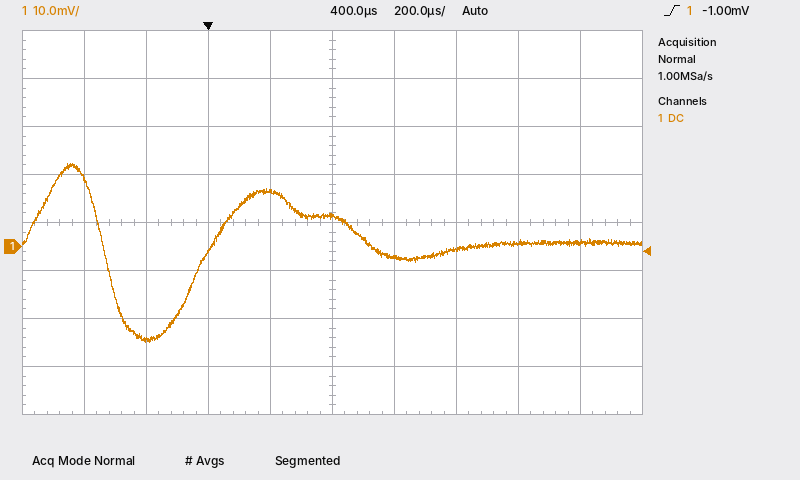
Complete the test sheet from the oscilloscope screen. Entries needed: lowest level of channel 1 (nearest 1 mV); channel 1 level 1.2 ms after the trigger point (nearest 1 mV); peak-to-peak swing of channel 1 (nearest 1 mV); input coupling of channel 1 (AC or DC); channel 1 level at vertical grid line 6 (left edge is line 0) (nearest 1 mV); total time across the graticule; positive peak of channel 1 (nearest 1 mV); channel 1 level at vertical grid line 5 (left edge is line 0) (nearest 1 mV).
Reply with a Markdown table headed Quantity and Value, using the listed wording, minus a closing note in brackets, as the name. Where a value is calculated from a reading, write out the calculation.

| Quantity | Value |
|---|---|
| lowest level of channel 1 | -20 mV |
| channel 1 level 1.2 ms after the trigger point | 1 mV |
| peak-to-peak swing of channel 1 | 17 mV − (-20 mV) = 37 mV |
| input coupling of channel 1 | DC |
| channel 1 level at vertical grid line 6 (left edge is line 0) | -2 mV |
| total time across the graticule | 2 ms |
| positive peak of channel 1 | 17 mV |
| channel 1 level at vertical grid line 5 (left edge is line 0) | 6 mV |
